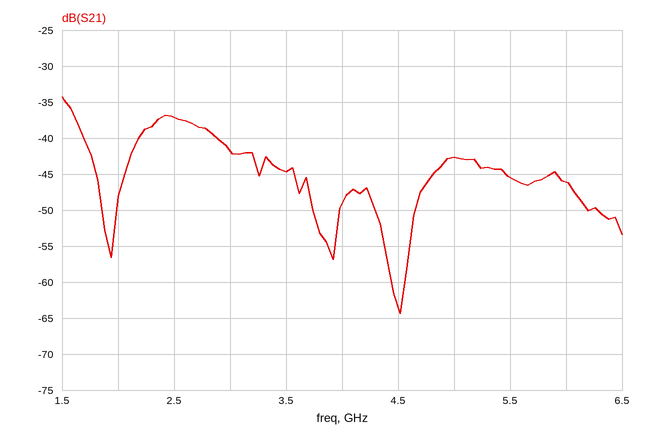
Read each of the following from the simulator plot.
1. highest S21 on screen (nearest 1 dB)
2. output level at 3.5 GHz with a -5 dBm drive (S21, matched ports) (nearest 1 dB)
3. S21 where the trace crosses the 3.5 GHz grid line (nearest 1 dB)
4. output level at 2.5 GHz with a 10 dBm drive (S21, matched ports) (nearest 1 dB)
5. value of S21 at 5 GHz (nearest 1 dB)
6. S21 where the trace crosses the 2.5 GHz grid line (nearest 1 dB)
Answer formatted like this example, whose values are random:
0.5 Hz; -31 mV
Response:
-34 dB; -50 dBm; -45 dB; -27 dBm; -43 dB; -37 dB
